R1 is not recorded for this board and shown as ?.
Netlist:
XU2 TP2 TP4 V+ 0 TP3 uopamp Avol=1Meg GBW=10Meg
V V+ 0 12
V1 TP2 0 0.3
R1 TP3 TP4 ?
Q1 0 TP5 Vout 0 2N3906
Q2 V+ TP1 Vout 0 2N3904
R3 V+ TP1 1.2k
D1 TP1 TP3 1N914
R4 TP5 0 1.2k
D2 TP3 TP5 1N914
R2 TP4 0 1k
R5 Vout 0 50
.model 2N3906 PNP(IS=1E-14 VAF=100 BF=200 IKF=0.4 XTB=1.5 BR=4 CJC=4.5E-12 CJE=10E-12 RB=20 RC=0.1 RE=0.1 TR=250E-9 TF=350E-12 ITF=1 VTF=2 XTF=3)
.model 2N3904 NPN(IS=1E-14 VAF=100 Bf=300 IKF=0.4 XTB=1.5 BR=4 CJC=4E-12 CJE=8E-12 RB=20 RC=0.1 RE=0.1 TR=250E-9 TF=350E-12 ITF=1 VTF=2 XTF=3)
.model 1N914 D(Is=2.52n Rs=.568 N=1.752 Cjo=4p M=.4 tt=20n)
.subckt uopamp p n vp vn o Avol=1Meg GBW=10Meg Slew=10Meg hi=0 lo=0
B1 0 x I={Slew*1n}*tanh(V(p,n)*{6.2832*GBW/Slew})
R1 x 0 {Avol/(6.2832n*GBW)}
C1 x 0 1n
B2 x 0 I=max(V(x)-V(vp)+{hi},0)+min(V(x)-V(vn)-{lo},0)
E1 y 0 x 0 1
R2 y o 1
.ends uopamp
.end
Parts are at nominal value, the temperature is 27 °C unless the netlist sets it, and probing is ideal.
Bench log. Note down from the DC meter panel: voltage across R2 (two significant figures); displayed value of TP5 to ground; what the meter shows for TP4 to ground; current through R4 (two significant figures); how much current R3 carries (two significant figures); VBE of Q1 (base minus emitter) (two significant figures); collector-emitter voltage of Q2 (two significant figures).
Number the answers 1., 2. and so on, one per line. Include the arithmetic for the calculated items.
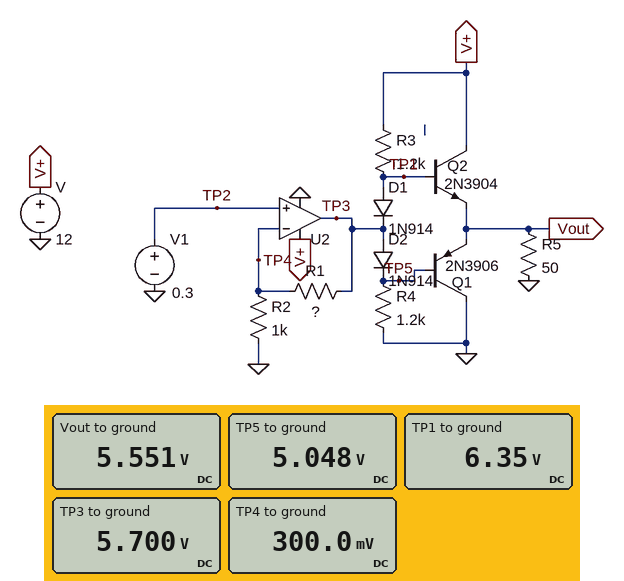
1. 300 mV = 300 mV
2. 5.048 V
3. 300.0 mV
4. (5.048 V) / 1.2 kΩ = 4.2 mA
5. (12 V - 6.35 V) / 1.2 kΩ = 4.7 mA
6. 5.048 V - 5.551 V = -500 mV
7. 12 V - 5.551 V = 6.4 V
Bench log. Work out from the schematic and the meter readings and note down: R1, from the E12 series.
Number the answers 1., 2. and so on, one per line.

1. 18 kΩ
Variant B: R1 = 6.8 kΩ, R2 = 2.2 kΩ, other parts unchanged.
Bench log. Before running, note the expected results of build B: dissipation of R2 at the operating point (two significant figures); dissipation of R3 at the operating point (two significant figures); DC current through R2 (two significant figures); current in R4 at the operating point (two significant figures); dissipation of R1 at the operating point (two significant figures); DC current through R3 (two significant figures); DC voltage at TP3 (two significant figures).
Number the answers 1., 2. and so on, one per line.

1. 41 µW
2. 85 mW
3. 140 µA
4. 560 µA
5. 130 µW
6. 8.4 mA
7. 1.2 V
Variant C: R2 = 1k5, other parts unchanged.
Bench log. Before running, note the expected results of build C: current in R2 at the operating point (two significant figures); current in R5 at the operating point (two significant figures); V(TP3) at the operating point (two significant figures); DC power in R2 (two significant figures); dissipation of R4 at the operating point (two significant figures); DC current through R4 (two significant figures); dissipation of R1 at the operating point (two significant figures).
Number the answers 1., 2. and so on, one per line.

1. 200 µA
2. 76 mA
3. 3.9 V
4. 60 µW
5. 8.9 mW
6. 2.7 mA
7. 720 µW
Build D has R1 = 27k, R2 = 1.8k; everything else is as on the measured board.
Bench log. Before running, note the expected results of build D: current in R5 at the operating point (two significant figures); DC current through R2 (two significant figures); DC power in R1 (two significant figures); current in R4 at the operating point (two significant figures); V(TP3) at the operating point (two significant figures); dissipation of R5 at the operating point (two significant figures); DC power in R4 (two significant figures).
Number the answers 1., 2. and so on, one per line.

1. 93 mA
2. 170 µA
3. 750 µW
4. 3.5 mA
5. 4.8 V
6. 440 mW
7. 14 mW
